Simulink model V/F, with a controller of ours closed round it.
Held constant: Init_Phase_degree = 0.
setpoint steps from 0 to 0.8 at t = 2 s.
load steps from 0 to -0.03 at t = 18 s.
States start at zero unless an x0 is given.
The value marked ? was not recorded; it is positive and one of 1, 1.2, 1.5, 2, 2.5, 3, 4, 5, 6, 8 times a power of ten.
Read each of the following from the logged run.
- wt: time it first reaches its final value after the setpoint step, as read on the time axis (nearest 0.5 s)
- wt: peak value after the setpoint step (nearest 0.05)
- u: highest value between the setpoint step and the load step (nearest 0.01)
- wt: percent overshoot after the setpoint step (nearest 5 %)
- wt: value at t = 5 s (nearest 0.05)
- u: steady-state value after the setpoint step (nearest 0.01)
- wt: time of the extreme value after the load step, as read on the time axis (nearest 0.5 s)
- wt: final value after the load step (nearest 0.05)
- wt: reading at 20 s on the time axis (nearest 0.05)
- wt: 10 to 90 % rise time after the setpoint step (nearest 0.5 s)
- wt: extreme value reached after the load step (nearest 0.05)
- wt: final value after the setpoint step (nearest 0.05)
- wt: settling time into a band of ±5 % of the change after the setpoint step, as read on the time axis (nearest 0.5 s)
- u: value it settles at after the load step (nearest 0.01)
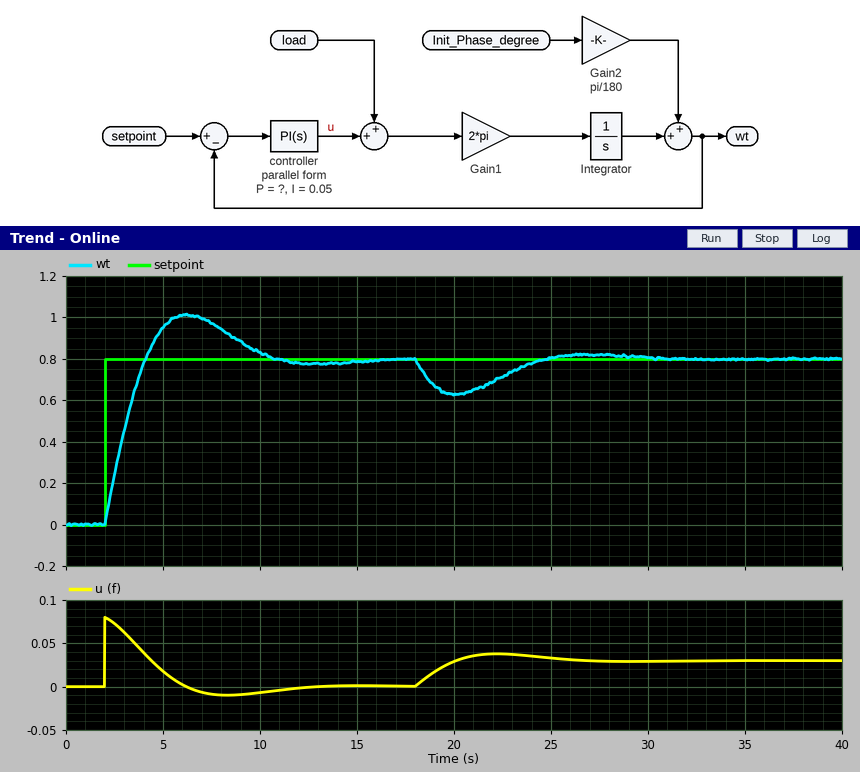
4.0 s
1.00
0.08
25 %
0.95
0.00
20.0 s
0.80
0.65
1.5 s
0.65
0.80
10.0 s
0.03
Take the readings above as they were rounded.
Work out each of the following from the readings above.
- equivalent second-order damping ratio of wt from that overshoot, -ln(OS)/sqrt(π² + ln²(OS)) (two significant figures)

0.40
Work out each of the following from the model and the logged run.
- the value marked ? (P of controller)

0.1
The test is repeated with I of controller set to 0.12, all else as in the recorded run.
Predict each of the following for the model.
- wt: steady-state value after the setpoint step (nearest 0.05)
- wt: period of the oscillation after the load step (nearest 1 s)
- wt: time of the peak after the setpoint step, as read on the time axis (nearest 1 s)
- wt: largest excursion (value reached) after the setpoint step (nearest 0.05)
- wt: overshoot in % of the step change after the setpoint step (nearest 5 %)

0.80
8 s
5 s
1.10
40 %
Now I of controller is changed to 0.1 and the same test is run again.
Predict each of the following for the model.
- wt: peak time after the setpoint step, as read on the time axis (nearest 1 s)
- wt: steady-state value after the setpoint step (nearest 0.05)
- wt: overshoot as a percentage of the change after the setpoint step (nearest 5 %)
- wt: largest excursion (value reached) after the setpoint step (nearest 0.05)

5 s
0.80
35 %
1.10
